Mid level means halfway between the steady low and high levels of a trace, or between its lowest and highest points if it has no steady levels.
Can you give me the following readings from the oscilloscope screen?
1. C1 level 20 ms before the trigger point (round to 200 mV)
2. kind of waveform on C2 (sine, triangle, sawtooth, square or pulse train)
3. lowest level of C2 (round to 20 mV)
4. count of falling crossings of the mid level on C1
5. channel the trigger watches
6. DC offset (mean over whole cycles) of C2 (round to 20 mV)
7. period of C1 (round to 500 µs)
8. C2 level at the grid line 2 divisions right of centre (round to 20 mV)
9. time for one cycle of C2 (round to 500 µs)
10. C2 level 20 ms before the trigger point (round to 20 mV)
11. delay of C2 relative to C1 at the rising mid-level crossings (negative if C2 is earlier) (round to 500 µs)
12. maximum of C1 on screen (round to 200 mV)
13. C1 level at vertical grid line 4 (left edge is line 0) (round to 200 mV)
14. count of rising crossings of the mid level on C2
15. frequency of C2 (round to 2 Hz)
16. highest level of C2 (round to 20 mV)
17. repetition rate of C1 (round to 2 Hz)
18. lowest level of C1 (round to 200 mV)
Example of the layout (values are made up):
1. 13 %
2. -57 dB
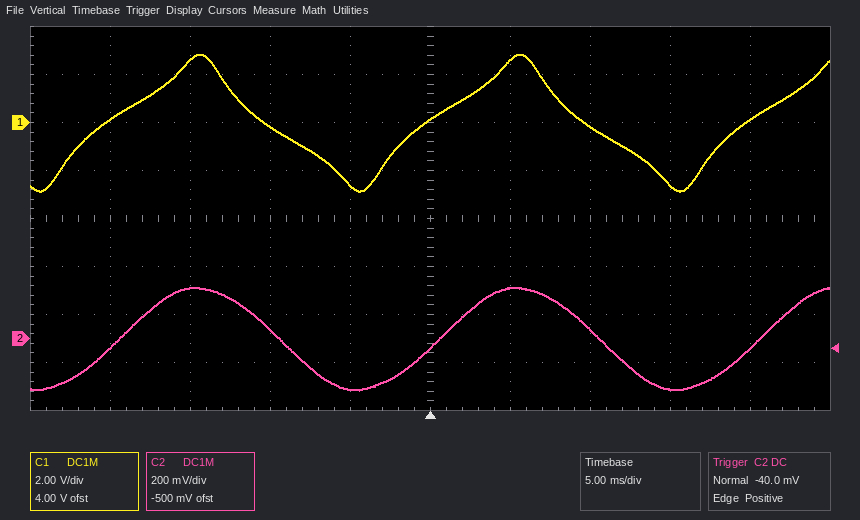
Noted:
1. 200 mV
2. sine
3. -220 mV
4. 2
5. C2
6. 0 mV
7. 20.0 ms
8. 40 mV
9. 20.0 ms
10. -40 mV
11. +1.0 ms
12. 2.8 V
13. -2.6 V
14. 3
15. 50 Hz
16. 220 mV
17. 50 Hz
18. -2.8 V
